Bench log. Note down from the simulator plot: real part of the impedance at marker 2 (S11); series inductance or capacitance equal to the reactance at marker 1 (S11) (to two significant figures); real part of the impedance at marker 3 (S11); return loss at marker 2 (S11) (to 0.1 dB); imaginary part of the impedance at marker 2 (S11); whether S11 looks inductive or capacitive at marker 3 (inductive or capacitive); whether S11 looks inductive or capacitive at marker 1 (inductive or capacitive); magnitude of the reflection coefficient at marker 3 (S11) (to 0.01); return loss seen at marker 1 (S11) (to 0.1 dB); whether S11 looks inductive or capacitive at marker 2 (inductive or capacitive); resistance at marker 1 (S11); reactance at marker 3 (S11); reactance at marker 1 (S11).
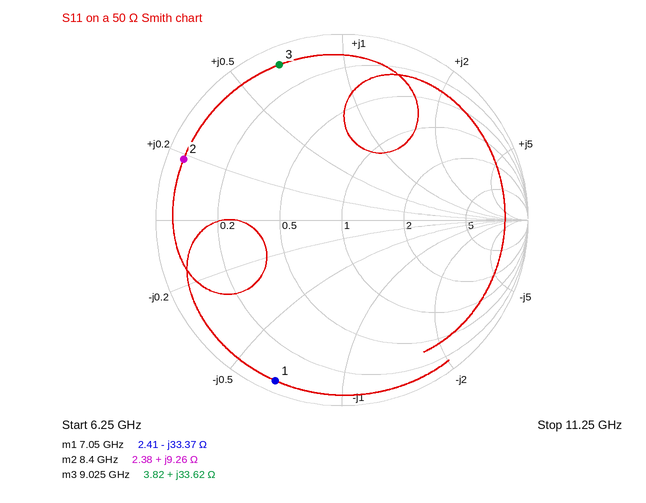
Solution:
2.38 Ω
680 fF
3.82 Ω
0.8 dB
+9.26 Ω
inductive
capacitive
0.90
0.6 dB
inductive
2.41 Ω
+33.62 Ω
-33.37 Ω
